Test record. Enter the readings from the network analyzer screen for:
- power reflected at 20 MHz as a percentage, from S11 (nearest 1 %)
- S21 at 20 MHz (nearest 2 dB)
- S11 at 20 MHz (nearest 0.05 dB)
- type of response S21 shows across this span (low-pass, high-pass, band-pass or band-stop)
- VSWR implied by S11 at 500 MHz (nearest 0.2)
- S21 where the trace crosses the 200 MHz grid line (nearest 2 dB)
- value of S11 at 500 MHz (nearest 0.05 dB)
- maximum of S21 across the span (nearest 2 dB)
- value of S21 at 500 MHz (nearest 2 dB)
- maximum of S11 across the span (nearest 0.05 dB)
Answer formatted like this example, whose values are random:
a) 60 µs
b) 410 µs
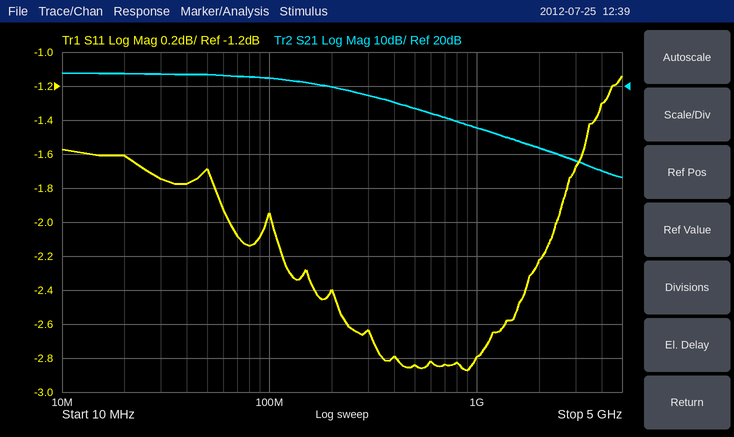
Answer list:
a) 69 %
b) 24 dB
c) -1.60 dB
d) low-pass
e) 6.2
f) 20 dB
g) -2.85 dB
h) 24 dB
i) 14 dB
j) -1.15 dB
